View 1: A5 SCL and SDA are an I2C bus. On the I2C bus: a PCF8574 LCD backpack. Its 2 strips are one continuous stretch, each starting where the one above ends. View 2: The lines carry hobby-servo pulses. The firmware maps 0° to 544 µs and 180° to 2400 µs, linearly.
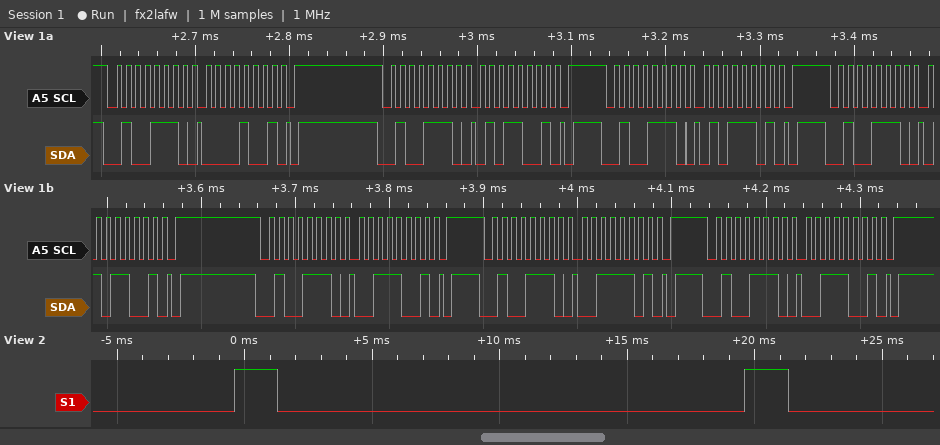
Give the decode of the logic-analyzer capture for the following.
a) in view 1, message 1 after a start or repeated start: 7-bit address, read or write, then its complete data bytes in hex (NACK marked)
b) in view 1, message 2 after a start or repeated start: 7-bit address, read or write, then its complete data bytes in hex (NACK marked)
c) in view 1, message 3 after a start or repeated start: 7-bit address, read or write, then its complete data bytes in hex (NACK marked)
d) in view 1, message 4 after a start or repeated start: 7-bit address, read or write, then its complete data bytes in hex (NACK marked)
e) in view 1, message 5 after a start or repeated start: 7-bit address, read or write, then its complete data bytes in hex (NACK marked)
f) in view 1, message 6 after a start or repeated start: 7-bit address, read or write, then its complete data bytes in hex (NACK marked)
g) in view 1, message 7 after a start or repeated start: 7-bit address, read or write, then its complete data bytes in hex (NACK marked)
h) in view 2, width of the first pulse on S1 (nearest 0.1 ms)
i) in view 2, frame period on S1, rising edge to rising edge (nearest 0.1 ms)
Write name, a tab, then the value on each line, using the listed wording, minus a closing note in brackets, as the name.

in view 1, message 1 after a start or repeated start: 7-bit address, read or write, then its complete data bytes in hex	0x27 write: 09
in view 1, message 2 after a start or repeated start: 7-bit address, read or write, then its complete data bytes in hex	0x27 write: 59
in view 1, message 3 after a start or repeated start: 7-bit address, read or write, then its complete data bytes in hex	0x27 write: 5D
in view 1, message 4 after a start or repeated start: 7-bit address, read or write, then its complete data bytes in hex	0x27 write: 59
in view 1, message 5 after a start or repeated start: 7-bit address, read or write, then its complete data bytes in hex	0x27 write: 39
in view 1, message 6 after a start or repeated start: 7-bit address, read or write, then its complete data bytes in hex	0x27 write: 3D
in view 1, message 7 after a start or repeated start: 7-bit address, read or write, then its complete data bytes in hex	0x27 write: 39
in view 2, width of the first pulse on S1	1.7 ms
in view 2, frame period on S1, rising edge to rising edge	20.0 ms
